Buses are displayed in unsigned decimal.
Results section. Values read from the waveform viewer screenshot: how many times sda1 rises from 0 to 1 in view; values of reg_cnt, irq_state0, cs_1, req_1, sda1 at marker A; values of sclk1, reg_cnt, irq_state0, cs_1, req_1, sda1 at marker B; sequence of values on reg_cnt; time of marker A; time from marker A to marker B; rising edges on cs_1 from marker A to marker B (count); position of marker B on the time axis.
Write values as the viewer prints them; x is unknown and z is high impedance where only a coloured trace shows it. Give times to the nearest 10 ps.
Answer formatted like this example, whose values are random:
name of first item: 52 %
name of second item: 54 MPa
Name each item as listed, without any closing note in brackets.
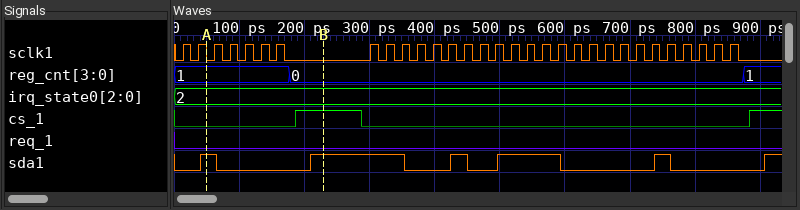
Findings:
how many times sda1 rises from 0 to 1 in view: 6
values of reg_cnt, irq_state0, cs_1, req_1, sda1 at marker A: reg_cnt=1, irq_state0=2, cs_1=0, req_1=0, sda1=1
values of sclk1, reg_cnt, irq_state0, cs_1, req_1, sda1 at marker B: sclk1=0, reg_cnt=0, irq_state0=2, cs_1=1, req_1=0, sda1=1
sequence of values on reg_cnt: 1, 0, 1
time of marker A: 50 ps
time from marker A to marker B: 180 ps
rising edges on cs_1 from marker A to marker B: 1
position of marker B on the time axis: 230 ps
